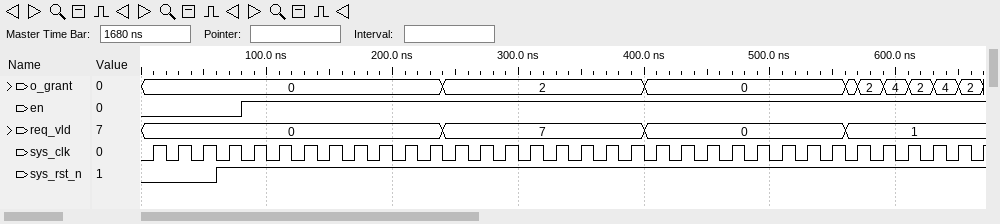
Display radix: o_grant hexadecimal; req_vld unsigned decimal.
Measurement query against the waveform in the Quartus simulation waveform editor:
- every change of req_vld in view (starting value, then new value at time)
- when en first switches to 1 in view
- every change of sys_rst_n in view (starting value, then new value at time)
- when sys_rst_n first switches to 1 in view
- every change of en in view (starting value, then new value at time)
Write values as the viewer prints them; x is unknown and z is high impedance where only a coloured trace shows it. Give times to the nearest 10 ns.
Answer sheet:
0, 7 at 240 ns, 0 at 400 ns, 1 at 560 ns
80 ns
0, 1 at 60 ns
60 ns
0, 1 at 80 ns
